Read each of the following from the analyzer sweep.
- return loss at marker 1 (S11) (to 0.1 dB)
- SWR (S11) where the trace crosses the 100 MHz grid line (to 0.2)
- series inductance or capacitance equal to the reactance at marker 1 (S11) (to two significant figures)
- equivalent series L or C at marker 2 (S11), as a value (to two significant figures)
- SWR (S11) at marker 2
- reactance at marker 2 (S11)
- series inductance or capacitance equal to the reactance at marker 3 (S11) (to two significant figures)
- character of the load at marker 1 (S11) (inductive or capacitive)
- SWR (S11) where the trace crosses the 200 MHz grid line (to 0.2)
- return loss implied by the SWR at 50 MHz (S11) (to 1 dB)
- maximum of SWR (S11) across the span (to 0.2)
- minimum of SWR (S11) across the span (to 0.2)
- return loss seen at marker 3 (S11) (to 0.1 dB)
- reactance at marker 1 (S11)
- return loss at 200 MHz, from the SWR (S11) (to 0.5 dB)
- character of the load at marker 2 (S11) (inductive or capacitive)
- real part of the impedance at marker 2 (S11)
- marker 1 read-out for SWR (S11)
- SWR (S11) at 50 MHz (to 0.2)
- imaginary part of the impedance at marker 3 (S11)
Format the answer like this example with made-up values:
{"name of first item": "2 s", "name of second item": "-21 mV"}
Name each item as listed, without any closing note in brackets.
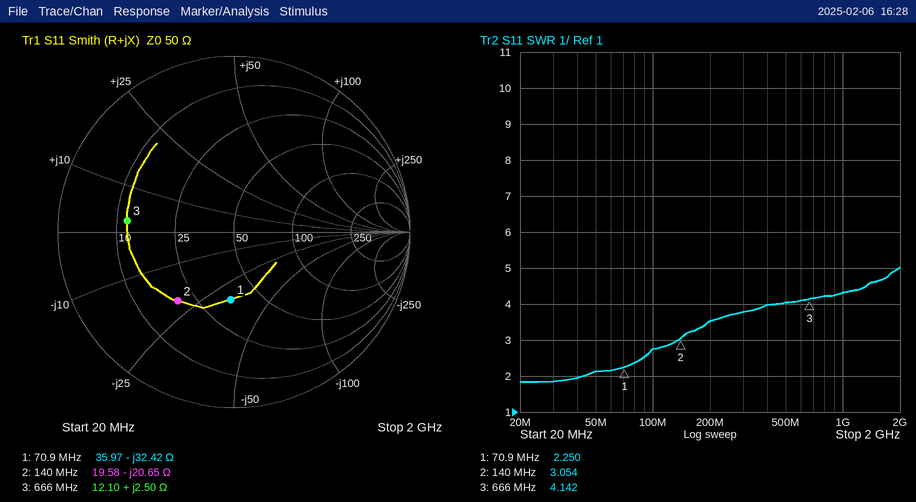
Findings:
{"return loss at marker 1 (S11)": "8.3 dB", "SWR (S11) where the trace crosses the 100 MHz grid line": "2.8", "series inductance or capacitance equal to the reactance at marker 1 (S11)": "69 pF", "equivalent series L or C at marker 2 (S11), as a value": "55 pF", "SWR (S11) at marker 2": "3.054", "reactance at marker 2": "-20.65 Ω", "series inductance or capacitance equal to the reactance at marker 3 (S11)": "600 pH", "character of the load at marker 1 (S11)": "capacitive", "SWR (S11) where the trace crosses the 200 MHz grid line": "3.6", "return loss implied by the SWR at 50 MHz (S11)": "9 dB", "maximum of SWR (S11) across the span": "5.0", "minimum of SWR (S11) across the span": "1.8", "return loss seen at marker 3 (S11)": "4.3 dB", "reactance at marker 1": "-32.42 Ω", "return loss at 200 MHz, from the SWR (S11)": "5.0 dB", "character of the load at marker 2 (S11)": "capacitive", "real part of the impedance at marker 2": "19.58 Ω", "marker 1 read-out for SWR": "2.250", "SWR (S11) at 50 MHz": "2.2", "imaginary part of the impedance at marker 3": "+2.50 Ω"}
